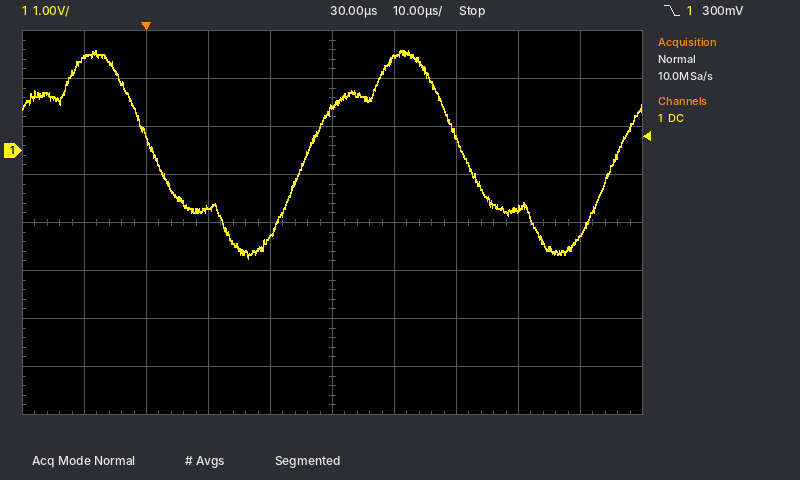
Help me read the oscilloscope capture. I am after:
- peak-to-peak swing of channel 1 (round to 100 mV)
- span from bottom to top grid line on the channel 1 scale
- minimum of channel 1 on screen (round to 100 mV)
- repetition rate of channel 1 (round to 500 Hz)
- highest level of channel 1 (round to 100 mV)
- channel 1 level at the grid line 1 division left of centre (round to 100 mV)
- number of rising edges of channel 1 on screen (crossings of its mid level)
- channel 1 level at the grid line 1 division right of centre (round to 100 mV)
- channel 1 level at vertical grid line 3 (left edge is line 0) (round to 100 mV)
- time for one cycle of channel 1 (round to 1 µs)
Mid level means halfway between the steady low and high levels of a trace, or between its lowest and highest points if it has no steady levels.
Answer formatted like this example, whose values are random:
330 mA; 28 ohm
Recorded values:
4.3 V; 8 V; -2.2 V; 20.0 kHz; 2.1 V; -1.8 V; 2; 1.9 V; -1.2 V; 50 µs
